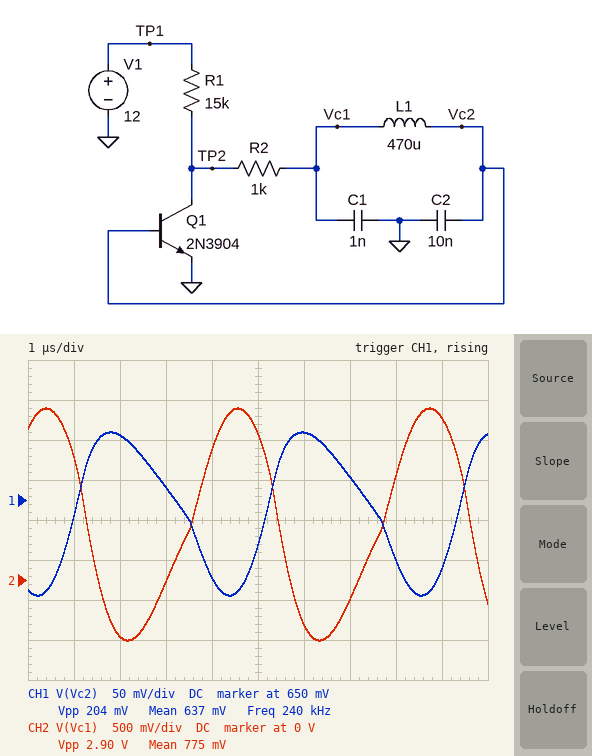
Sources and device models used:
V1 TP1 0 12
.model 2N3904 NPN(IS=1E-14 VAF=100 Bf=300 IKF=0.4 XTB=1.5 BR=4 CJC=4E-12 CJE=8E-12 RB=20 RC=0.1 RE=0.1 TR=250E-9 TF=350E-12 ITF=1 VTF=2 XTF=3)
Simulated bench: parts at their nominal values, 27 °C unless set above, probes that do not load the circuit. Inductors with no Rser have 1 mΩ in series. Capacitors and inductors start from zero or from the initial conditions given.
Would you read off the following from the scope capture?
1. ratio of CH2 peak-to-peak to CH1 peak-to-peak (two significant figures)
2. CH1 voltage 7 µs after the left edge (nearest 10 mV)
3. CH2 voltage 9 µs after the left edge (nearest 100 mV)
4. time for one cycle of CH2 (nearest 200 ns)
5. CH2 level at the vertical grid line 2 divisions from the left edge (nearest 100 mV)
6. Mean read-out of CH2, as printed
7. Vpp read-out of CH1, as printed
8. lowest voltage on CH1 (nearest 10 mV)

14
680 mV
2.0 V
4.2 µs
-700 mV
775 mV
204 mV
530 mV
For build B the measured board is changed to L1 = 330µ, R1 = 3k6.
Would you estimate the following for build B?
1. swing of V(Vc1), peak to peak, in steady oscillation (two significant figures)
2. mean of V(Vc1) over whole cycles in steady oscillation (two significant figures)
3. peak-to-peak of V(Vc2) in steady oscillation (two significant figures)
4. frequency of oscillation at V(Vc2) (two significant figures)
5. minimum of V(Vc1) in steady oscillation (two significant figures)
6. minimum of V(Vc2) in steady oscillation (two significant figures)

5.3 V
680 mV
300 mV
290 kHz
-1.8 V
520 mV
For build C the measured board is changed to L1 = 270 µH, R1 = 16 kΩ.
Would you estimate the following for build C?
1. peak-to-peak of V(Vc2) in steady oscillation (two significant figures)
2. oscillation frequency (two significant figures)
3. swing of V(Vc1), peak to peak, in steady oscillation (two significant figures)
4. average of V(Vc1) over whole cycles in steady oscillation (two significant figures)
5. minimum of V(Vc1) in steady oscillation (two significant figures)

210 mV
310 kHz
2.8 V
640 mV
-720 mV
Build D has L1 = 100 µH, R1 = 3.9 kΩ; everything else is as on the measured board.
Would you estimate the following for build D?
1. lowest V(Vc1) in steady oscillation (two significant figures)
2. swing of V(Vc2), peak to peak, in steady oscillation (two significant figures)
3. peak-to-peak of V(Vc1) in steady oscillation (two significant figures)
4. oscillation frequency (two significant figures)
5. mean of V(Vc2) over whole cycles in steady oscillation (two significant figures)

-1.5 V
320 mV
4.4 V
510 kHz
670 mV
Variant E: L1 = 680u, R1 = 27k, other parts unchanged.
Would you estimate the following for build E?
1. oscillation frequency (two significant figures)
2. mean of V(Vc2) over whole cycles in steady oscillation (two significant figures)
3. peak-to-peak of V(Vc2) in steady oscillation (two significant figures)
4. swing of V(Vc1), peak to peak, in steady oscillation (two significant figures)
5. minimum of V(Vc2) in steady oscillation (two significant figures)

200 kHz
630 mV
180 mV
2.4 V
530 mV
